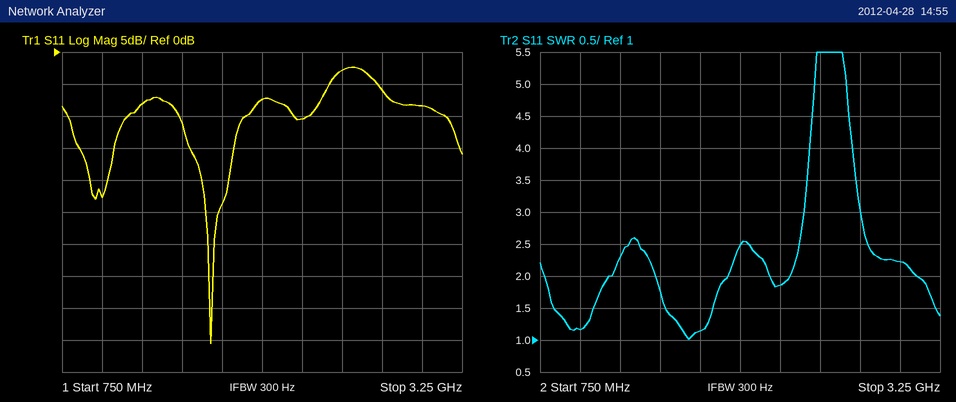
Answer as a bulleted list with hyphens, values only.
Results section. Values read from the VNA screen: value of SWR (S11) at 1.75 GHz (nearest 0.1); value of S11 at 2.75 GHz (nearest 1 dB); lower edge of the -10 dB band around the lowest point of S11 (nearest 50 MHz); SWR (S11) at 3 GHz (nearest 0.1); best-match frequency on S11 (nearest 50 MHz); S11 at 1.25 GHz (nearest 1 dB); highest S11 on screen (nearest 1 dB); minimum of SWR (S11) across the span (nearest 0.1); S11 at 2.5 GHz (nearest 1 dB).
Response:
- 1.1
- -6 dB
- 1.50 GHz
- 2.2
- 1.70 GHz
- -8 dB
- -2 dB
- 1.0
- -3 dB
